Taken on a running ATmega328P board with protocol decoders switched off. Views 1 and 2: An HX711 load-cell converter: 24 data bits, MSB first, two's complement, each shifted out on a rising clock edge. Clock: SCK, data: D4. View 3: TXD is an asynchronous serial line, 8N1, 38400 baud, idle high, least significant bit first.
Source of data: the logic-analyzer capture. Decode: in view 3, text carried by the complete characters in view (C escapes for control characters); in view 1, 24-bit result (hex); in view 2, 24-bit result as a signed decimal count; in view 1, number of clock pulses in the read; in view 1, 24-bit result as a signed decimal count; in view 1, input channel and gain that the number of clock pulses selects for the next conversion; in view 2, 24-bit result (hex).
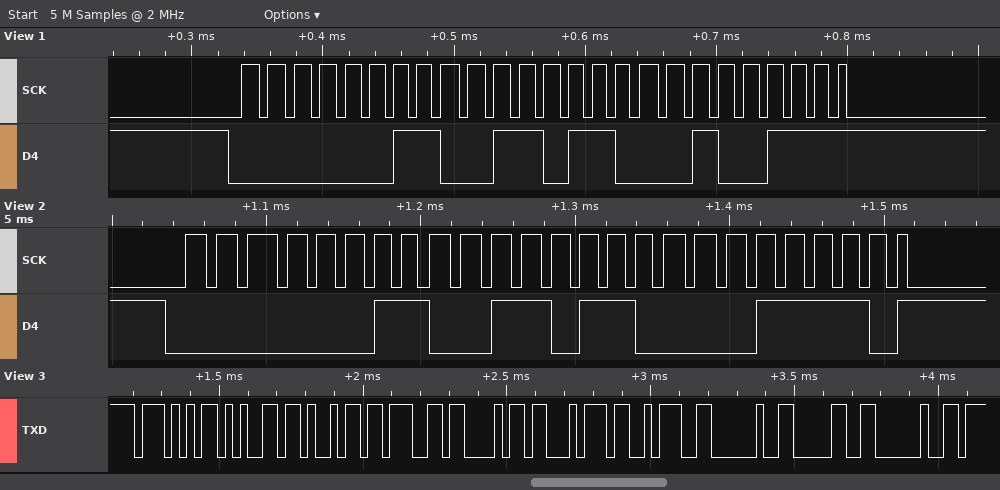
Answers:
"Weight: 0 "
0x033627
210462
25
210471
channel A, gain 128
0x03361E
